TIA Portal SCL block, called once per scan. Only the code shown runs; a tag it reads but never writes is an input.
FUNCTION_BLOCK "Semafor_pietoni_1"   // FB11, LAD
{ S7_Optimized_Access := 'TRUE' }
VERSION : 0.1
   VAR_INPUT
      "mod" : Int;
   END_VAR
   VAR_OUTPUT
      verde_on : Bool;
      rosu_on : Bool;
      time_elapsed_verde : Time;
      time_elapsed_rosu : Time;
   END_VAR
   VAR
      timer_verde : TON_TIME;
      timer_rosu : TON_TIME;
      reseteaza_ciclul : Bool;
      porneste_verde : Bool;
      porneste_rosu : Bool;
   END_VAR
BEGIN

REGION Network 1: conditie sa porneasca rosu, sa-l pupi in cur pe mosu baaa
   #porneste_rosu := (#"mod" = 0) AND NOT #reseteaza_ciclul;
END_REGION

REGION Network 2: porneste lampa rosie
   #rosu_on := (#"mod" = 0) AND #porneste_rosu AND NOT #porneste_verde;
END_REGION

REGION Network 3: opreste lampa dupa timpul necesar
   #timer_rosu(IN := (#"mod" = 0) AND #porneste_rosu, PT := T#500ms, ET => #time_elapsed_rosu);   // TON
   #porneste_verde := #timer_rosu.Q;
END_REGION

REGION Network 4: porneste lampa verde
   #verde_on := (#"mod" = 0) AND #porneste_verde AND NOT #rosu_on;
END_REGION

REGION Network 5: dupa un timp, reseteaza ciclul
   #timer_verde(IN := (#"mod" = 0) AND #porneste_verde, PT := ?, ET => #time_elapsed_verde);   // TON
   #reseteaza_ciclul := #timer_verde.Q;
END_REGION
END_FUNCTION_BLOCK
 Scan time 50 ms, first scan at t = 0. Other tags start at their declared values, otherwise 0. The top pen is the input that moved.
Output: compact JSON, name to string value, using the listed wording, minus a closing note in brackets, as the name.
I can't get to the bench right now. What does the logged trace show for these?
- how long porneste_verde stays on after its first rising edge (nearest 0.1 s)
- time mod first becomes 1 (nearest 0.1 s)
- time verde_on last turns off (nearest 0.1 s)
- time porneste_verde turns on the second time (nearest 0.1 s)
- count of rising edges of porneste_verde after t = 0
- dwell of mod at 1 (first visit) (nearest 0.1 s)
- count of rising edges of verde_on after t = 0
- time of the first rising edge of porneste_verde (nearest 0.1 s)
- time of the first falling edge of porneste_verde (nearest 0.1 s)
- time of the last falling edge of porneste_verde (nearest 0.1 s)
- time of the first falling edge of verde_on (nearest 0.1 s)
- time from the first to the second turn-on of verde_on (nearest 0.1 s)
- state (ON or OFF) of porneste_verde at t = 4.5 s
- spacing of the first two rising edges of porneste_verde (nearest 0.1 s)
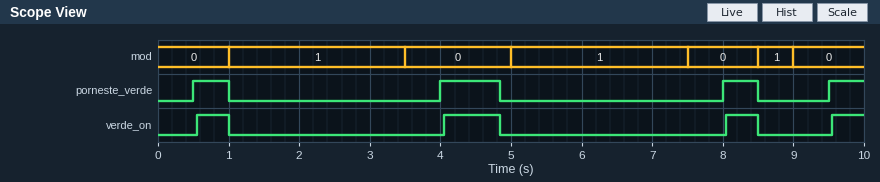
{"how long porneste_verde stays on after its first rising edge": "0.5 s", "time mod first becomes 1": "1.0 s", "time verde_on last turns off": "8.5 s", "time porneste_verde turns on the second time": "4.0 s", "count of rising edges of porneste_verde after t = 0": "4", "dwell of mod at 1 (first visit)": "2.5 s", "count of rising edges of verde_on after t = 0": "4", "time of the first rising edge of porneste_verde": "0.5 s", "time of the first falling edge of porneste_verde": "1.0 s", "time of the last falling edge of porneste_verde": "8.5 s", "time of the first falling edge of verde_on": "1.0 s", "time from the first to the second turn-on of verde_on": "3.5 s", "state (ON or OFF) of porneste_verde at t = 4.5 s": "ON", "spacing of the first two rising edges of porneste_verde": "3.5 s"}
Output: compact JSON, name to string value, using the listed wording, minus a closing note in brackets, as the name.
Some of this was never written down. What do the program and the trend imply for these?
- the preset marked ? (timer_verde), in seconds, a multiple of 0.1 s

{"the preset marked ? (timer_verde), in seconds, a multiple of 0.1 s": "0.8 s"}
